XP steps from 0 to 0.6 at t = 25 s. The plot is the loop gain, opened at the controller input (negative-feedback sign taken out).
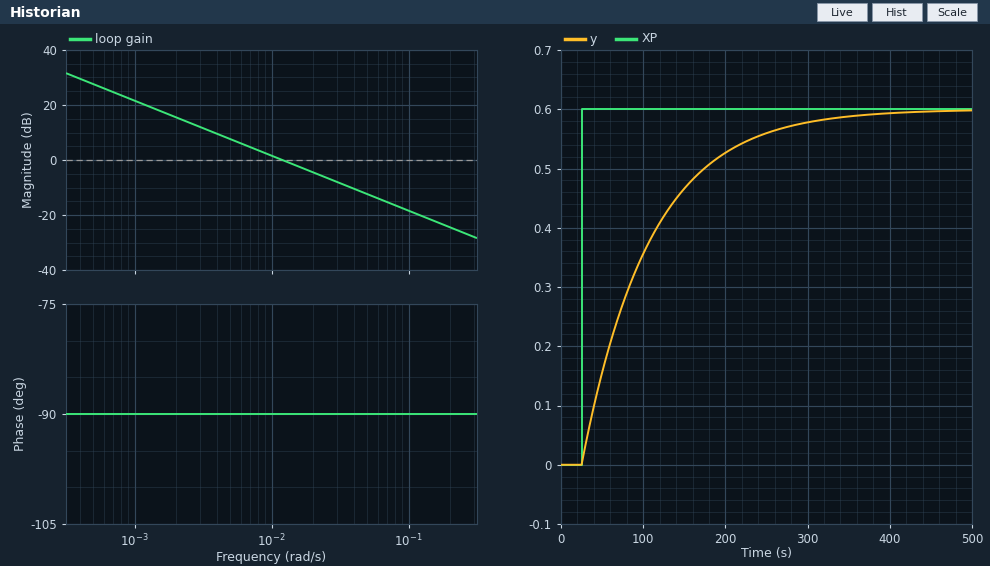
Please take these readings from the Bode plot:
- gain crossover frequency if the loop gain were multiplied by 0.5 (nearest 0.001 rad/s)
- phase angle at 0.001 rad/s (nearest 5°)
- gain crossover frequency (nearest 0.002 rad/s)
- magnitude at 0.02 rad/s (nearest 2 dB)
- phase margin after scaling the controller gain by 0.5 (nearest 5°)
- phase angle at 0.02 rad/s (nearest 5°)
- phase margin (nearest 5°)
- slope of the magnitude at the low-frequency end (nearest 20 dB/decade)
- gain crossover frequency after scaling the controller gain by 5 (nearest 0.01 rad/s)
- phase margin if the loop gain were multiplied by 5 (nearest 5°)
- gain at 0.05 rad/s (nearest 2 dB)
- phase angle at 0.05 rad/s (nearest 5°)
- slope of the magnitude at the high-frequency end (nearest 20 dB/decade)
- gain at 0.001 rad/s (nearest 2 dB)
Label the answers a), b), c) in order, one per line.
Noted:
a) 0.006 rad/s
b) -90°
c) 0.012 rad/s
d) -4 dB
e) 90°
f) -90°
g) 90°
h) -20 dB/decade
i) 0.06 rad/s
j) 90°
k) -12 dB
l) -90°
m) -20 dB/decade
n) 22 dB
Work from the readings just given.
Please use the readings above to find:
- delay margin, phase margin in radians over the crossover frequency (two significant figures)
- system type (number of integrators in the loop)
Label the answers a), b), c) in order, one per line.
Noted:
a) 130 s
b) 1
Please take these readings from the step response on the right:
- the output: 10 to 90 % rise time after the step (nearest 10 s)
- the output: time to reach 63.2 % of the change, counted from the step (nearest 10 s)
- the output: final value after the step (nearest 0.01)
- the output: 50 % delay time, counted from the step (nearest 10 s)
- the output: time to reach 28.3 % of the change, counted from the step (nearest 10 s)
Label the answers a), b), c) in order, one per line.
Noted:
a) 180 s
b) 80 s
c) 0.60
d) 60 s
e) 30 s
